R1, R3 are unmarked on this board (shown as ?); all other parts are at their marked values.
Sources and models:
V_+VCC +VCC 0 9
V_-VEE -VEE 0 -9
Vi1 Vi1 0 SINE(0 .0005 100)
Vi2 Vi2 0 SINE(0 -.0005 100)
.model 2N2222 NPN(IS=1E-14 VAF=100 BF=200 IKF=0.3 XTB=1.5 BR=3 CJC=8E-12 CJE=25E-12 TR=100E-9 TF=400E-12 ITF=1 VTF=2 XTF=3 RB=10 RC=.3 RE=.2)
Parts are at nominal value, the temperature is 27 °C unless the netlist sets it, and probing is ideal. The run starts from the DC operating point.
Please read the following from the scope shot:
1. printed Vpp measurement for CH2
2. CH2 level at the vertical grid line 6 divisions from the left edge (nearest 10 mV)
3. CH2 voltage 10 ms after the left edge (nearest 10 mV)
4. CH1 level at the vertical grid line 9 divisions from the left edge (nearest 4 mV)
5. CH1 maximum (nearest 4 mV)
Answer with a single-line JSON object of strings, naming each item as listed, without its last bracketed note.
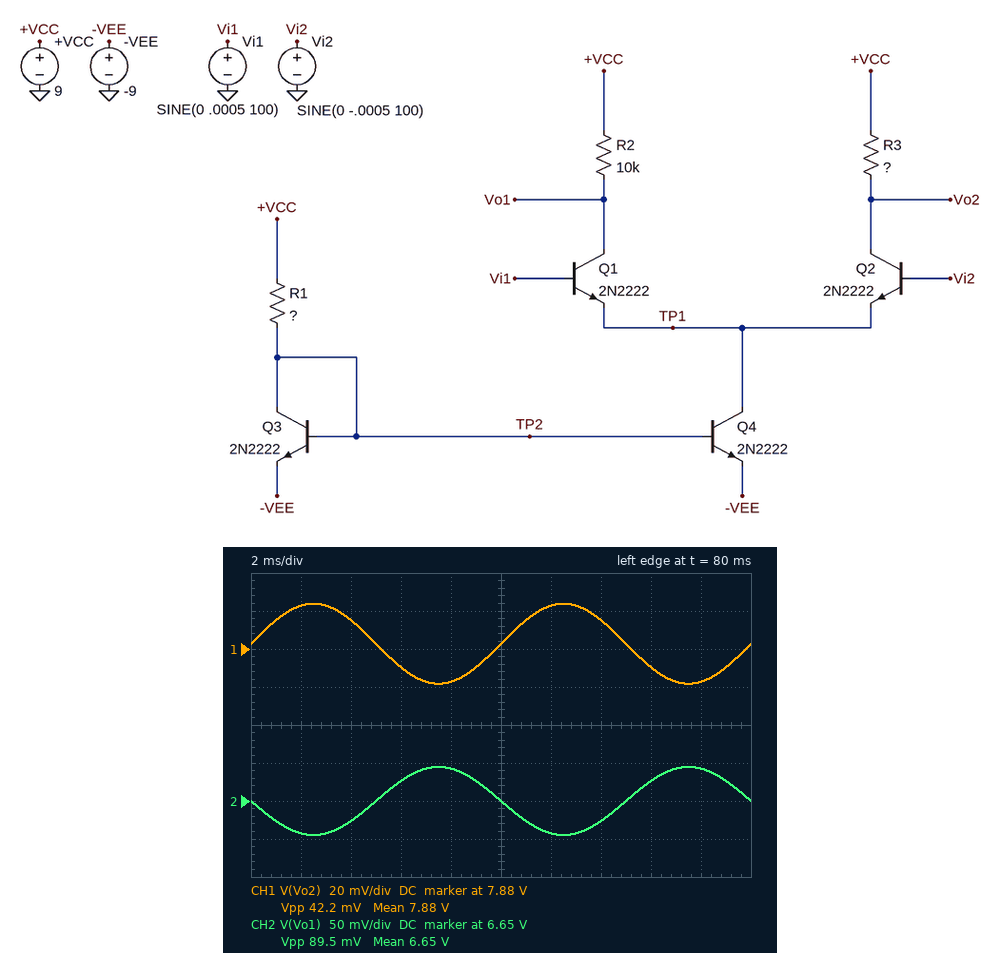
{"printed Vpp measurement for CH2": "89.5 mV", "CH2 level at the vertical grid line 6 divisions from the left edge": "6.61 V", "CH2 voltage 10 ms after the left edge": "6.65 V", "CH1 level at the vertical grid line 9 divisions from the left edge": "7.864 V", "CH1 maximum": "7.904 V"}
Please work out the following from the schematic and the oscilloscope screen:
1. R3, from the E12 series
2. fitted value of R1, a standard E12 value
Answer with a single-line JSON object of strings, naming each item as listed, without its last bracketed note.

{"R3, from the E12 series": "4.7 kΩ", "fitted value of R1, a standard E12 value": "39 kΩ"}
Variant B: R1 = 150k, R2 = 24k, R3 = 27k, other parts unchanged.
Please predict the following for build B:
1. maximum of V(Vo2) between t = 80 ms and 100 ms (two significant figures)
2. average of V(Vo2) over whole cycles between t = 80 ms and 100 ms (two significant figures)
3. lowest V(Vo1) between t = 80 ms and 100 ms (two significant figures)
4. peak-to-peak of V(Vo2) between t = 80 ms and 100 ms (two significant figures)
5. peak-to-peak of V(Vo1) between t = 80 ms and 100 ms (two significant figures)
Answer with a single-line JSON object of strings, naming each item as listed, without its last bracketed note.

{"maximum of V(Vo2) between t = 80 ms and 100 ms": "7.4 V", "average of V(Vo2) over whole cycles between t = 80 ms and 100 ms": "7.3 V", "lowest V(Vo1) between t = 80 ms and 100 ms": "7.5 V", "peak-to-peak of V(Vo2) between t = 80 ms and 100 ms": "63 mV", "peak-to-peak of V(Vo1) between t = 80 ms and 100 ms": "56 mV"}
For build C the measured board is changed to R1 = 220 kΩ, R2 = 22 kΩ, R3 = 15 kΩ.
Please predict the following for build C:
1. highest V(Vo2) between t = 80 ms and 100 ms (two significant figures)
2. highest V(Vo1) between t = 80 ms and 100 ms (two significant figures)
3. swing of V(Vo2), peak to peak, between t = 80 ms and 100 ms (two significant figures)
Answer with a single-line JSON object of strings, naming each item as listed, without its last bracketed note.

{"highest V(Vo2) between t = 80 ms and 100 ms": "8.4 V", "highest V(Vo1) between t = 80 ms and 100 ms": "8.1 V", "swing of V(Vo2), peak to peak, between t = 80 ms and 100 ms": "24 mV"}
